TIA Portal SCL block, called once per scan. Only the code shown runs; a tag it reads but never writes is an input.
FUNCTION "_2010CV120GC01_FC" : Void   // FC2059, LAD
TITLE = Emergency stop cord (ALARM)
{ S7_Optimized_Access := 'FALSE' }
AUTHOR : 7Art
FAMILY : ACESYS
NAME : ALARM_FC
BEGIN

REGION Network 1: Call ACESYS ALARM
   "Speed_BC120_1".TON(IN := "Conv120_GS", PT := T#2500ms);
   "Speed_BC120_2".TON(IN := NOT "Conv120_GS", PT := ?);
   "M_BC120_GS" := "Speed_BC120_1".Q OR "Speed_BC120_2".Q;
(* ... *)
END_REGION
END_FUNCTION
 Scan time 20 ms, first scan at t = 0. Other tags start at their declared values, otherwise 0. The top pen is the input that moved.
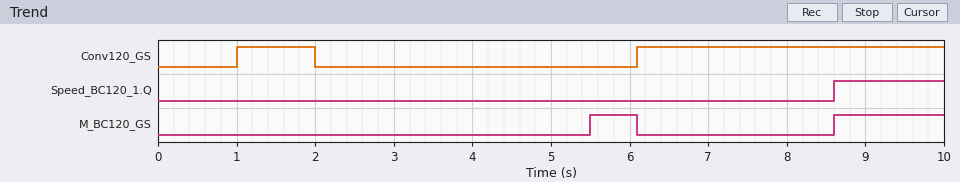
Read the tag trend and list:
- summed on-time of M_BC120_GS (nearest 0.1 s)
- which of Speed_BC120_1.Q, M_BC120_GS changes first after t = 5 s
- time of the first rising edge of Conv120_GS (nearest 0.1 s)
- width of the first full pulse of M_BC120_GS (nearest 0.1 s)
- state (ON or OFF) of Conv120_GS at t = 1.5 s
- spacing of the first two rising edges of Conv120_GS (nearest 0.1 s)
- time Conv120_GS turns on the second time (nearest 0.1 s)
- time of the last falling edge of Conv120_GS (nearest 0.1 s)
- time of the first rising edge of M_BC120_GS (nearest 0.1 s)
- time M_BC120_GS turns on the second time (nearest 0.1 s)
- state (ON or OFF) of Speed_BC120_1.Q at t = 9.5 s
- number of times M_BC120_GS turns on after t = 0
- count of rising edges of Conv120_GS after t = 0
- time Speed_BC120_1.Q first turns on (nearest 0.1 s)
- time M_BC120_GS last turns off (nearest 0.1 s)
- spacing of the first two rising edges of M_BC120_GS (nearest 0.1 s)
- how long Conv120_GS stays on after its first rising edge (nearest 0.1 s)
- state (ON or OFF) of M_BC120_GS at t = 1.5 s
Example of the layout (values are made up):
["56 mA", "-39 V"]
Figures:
["2.0 s", "M_BC120_GS", "1.0 s", "0.6 s", "ON", "5.1 s", "6.1 s", "2.0 s", "5.5 s", "8.6 s", "ON", "2", "2", "8.6 s", "6.1 s", "3.1 s", "1.0 s", "OFF"]
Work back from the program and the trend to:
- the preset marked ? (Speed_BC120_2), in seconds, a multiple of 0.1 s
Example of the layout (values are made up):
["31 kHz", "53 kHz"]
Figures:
["3.5 s"]
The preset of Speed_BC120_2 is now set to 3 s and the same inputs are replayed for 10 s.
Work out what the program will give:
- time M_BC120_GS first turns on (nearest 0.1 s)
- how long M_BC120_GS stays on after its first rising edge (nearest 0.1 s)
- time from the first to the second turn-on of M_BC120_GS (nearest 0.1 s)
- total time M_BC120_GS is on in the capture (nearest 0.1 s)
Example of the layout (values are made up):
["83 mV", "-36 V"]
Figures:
["5.0 s", "1.1 s", "3.6 s", "2.5 s"]
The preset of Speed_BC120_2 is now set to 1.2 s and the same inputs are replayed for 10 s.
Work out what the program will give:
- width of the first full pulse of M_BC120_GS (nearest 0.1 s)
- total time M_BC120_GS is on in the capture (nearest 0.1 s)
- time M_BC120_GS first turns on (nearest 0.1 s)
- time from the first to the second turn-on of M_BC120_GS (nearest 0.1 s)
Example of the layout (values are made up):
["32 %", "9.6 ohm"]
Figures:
["2.9 s", "4.3 s", "3.2 s", "5.4 s"]
